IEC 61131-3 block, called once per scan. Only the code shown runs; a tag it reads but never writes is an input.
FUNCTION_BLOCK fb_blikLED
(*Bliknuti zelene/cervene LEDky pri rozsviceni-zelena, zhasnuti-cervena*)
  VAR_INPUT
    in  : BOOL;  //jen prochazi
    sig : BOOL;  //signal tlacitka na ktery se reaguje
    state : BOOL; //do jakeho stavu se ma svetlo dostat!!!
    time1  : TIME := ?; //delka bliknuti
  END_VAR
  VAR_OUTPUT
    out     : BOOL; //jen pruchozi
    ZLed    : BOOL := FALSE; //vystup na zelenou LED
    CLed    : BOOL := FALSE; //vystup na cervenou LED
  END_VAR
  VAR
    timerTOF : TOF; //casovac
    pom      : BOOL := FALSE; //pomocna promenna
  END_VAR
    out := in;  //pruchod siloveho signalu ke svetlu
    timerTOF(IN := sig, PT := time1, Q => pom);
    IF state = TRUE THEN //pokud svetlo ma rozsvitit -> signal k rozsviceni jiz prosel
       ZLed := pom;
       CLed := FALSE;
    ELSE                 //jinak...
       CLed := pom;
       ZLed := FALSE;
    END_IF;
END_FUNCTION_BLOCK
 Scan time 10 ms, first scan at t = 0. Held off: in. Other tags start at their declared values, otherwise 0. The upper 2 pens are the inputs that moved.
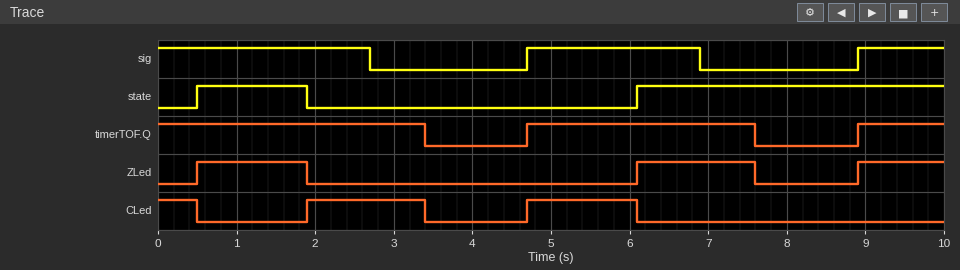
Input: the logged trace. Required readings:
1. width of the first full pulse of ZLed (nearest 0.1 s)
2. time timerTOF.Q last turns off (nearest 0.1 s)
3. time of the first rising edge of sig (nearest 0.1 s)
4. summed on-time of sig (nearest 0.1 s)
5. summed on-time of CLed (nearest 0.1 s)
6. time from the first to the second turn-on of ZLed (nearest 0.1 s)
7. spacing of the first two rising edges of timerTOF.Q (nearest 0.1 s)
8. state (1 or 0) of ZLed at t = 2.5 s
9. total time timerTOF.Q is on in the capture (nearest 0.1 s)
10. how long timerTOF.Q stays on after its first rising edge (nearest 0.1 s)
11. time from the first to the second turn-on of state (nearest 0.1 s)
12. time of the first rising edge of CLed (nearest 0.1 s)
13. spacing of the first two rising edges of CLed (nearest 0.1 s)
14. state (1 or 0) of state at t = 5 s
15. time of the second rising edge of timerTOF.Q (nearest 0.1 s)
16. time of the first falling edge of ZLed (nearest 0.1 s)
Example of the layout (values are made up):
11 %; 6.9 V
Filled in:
1.4 s; 7.6 s; 4.7 s; 6.0 s; 3.4 s; 5.6 s; 4.2 s; 0; 7.4 s; 2.9 s; 5.6 s; 1.9 s; 2.8 s; 0; 8.9 s; 1.9 s
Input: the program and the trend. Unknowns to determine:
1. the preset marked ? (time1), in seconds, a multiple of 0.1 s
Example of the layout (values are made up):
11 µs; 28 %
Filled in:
0.7 s
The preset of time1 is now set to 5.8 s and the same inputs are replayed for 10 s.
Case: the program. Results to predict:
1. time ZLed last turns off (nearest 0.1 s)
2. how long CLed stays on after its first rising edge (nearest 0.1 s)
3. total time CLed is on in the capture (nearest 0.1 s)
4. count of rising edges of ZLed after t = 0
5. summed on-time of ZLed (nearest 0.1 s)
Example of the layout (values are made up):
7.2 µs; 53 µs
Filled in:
1.9 s; 4.2 s; 4.7 s; 2; 5.3 s
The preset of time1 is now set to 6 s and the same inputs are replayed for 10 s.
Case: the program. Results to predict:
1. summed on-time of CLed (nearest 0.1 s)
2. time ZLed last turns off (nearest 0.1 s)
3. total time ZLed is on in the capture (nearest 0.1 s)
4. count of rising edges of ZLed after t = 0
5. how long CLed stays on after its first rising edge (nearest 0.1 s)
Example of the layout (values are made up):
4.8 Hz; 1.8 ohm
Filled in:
4.7 s; 1.9 s; 5.3 s; 2; 4.2 s
